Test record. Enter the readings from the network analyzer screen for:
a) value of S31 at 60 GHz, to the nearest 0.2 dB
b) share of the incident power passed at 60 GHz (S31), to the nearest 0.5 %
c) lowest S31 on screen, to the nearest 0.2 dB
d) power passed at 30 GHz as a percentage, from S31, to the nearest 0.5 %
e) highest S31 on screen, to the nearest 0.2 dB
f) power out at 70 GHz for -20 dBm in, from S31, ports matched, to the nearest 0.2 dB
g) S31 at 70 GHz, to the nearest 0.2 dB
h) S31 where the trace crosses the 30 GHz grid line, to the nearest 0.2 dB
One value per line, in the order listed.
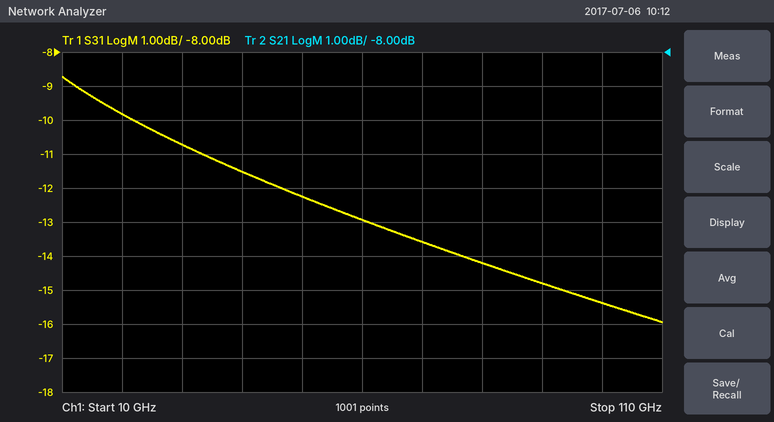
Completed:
-13.0 dB
5.0 %
-16.0 dB
8.5 %
-8.8 dB
-33.6 dBm
-13.6 dB
-10.8 dB
